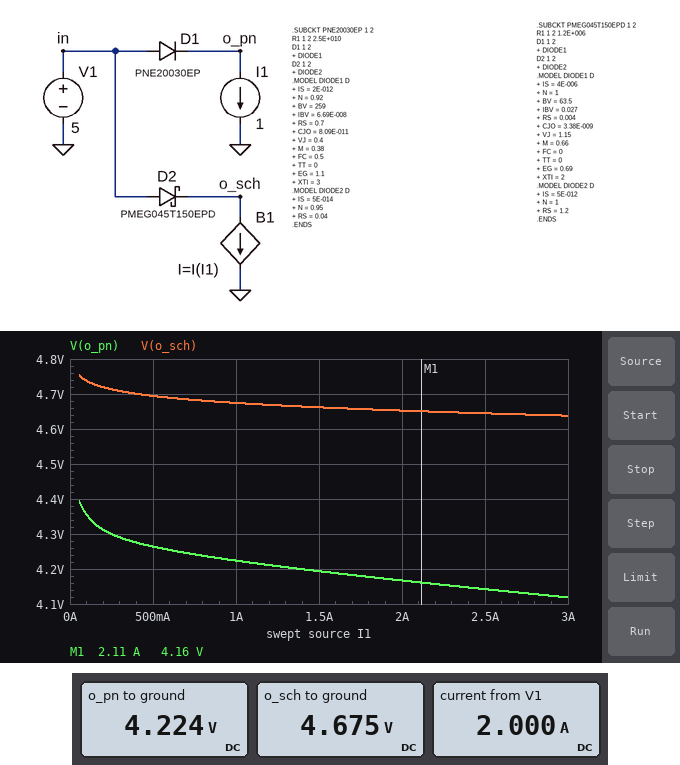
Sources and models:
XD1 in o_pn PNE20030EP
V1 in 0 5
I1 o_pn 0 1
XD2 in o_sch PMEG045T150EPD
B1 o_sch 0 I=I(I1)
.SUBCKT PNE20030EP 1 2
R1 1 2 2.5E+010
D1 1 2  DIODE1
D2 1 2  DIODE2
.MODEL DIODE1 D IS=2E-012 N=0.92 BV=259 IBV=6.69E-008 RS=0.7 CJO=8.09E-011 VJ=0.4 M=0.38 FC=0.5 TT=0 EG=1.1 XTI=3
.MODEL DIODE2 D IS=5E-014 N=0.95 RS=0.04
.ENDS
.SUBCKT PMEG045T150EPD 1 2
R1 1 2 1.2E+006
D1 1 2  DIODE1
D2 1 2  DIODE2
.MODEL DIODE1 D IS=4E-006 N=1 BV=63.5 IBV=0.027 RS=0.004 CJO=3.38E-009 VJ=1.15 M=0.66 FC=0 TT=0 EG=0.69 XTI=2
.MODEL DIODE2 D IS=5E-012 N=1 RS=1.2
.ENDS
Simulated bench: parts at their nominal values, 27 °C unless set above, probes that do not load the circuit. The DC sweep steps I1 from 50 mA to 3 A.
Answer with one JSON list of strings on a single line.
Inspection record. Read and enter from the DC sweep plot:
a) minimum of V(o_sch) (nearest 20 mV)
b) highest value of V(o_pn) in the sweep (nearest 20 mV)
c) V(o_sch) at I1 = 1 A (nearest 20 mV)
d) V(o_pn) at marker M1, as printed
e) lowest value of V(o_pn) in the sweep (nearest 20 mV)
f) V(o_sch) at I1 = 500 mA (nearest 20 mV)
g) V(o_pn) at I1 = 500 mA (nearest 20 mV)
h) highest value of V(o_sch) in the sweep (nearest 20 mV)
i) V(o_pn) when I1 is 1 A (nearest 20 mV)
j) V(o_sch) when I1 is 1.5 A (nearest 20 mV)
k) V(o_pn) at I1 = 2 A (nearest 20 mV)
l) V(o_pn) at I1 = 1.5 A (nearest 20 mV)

["4.64 V", "4.40 V", "4.68 V", "4.16 V", "4.12 V", "4.70 V", "4.26 V", "4.76 V", "4.22 V", "4.66 V", "4.16 V", "4.20 V"]
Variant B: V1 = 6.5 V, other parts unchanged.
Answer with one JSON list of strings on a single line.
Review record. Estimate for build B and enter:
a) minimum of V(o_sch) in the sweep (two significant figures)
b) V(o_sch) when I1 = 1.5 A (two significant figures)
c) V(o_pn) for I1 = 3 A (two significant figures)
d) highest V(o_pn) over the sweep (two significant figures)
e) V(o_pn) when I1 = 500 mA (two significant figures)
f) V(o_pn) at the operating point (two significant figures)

["6.1 V", "6.2 V", "5.6 V", "5.9 V", "5.8 V", "5.7 V"]
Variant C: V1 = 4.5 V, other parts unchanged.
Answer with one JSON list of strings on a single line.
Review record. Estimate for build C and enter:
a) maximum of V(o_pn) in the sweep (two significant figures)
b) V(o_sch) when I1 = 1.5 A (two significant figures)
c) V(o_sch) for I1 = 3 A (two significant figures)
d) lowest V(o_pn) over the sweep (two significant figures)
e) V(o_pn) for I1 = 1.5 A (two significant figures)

["3.9 V", "4.2 V", "4.1 V", "3.6 V", "3.7 V"]
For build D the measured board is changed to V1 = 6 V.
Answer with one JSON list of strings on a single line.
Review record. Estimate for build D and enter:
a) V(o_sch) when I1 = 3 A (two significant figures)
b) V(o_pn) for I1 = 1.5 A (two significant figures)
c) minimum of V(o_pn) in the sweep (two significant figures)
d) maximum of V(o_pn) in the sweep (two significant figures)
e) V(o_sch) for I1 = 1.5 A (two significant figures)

["5.6 V", "5.2 V", "5.1 V", "5.4 V", "5.7 V"]
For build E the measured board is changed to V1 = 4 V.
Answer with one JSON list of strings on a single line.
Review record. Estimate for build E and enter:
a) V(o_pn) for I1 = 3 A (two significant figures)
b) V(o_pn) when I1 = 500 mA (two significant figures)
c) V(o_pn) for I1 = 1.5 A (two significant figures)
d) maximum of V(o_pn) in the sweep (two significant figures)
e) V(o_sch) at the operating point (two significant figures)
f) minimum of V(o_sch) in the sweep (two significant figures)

["3.1 V", "3.3 V", "3.2 V", "3.4 V", "3.7 V", "3.6 V"]
